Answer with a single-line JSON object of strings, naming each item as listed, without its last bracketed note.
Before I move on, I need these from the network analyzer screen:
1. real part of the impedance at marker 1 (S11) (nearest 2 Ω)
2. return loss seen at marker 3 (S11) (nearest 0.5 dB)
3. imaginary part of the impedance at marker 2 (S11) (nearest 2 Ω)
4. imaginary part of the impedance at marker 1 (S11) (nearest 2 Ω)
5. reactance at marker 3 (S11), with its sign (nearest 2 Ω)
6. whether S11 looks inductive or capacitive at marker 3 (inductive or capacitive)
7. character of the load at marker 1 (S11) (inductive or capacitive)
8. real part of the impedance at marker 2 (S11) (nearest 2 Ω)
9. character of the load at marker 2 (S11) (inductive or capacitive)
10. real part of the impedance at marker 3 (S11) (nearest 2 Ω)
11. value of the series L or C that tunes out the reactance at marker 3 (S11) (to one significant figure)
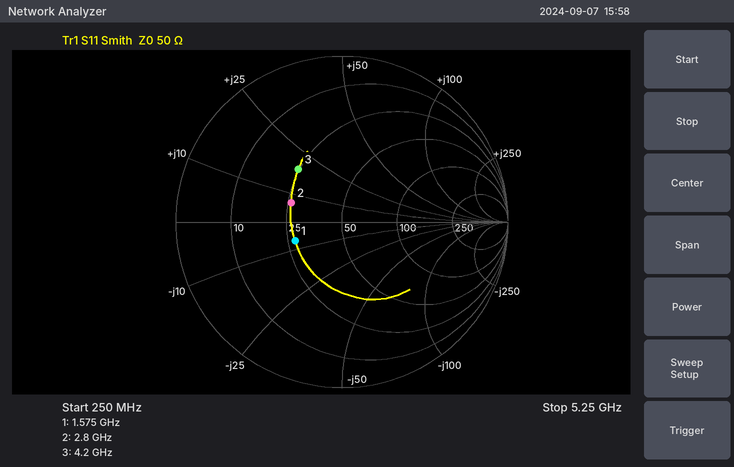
{"real part of the impedance at marker 1 (S11)": "28 Ω", "return loss seen at marker 3 (S11)": "7.5 dB", "imaginary part of the impedance at marker 2 (S11)": "+6 Ω", "imaginary part of the impedance at marker 1 (S11)": "-6 Ω", "reactance at marker 3 (S11), with its sign": "+18 Ω", "whether S11 looks inductive or capacitive at marker 3": "inductive", "character of the load at marker 1 (S11)": "capacitive", "real part of the impedance at marker 2 (S11)": "26 Ω", "character of the load at marker 2 (S11)": "inductive", "real part of the impedance at marker 3 (S11)": "24 Ω", "value of the series L or C that tunes out the reactance at marker 3 (S11)": "2 pF"}
